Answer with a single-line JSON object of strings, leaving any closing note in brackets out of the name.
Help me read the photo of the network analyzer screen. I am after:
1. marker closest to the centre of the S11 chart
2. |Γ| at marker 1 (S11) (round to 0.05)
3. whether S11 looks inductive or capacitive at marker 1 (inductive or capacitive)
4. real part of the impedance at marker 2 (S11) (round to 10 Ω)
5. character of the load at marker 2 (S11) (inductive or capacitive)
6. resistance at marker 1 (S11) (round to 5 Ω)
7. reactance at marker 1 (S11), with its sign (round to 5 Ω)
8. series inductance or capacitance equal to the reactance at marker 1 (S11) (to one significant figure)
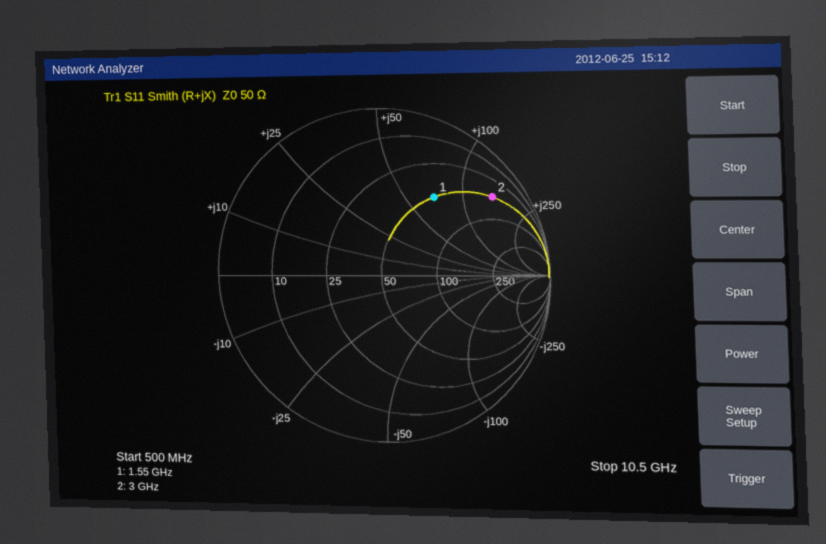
{"marker closest to the centre of the S11 chart": "marker 1", "|Γ| at marker 1 (S11)": "0.55", "whether S11 looks inductive or capacitive at marker 1": "inductive", "real part of the impedance at marker 2 (S11)": "50 Ω", "character of the load at marker 2 (S11)": "inductive", "resistance at marker 1 (S11)": "50 Ω", "reactance at marker 1 (S11), with its sign": "+70 Ω", "series inductance or capacitance equal to the reactance at marker 1 (S11)": "7 nH"}
